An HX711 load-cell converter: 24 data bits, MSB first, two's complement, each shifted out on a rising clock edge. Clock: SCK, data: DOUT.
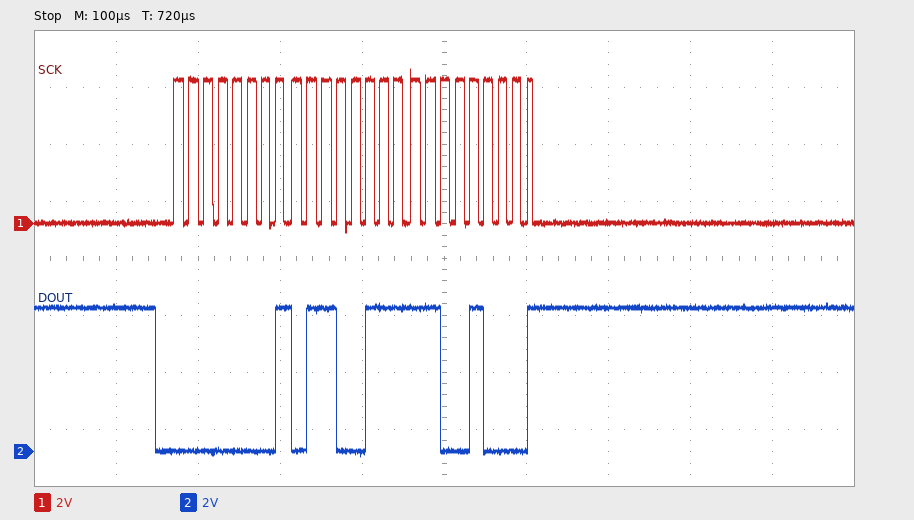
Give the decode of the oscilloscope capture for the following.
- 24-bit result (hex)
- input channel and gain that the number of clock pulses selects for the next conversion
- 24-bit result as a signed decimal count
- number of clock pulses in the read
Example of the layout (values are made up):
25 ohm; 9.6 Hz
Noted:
0x0167C8; channel A, gain 128; 92104; 25
